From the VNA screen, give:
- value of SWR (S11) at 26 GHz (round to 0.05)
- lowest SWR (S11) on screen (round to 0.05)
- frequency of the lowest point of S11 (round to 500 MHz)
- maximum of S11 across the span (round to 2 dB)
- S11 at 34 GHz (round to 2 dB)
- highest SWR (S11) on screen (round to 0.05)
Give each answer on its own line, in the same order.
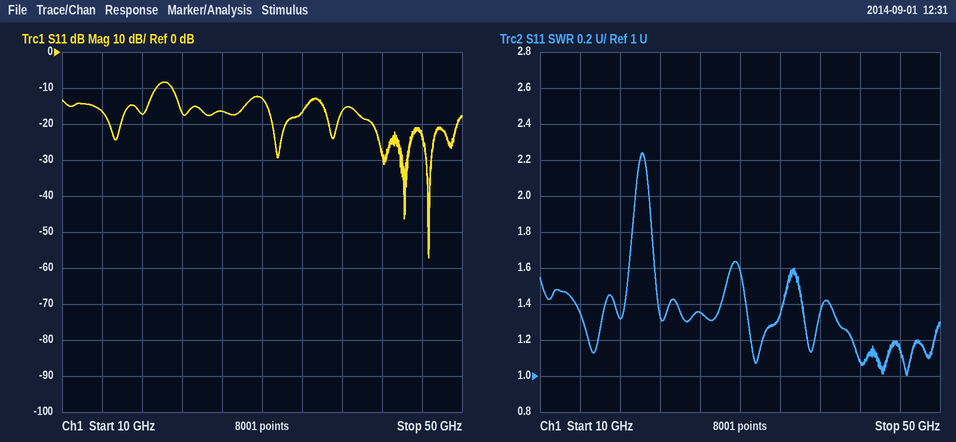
1.35
1.00
46.5 GHz
-8 dB
-16 dB
2.25
